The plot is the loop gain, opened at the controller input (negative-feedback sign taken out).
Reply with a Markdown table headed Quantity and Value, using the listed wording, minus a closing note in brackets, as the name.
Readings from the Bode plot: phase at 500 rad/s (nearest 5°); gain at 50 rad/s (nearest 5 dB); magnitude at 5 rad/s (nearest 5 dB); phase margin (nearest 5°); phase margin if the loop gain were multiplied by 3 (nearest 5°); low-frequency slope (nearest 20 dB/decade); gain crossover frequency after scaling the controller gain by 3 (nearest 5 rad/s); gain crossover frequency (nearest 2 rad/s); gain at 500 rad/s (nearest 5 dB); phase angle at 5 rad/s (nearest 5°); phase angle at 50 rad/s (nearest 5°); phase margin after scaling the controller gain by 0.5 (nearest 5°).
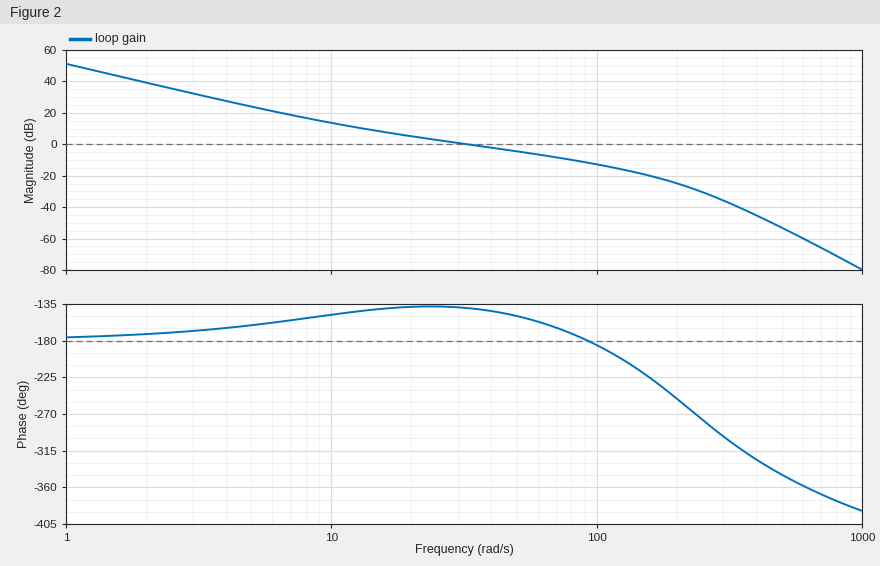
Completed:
| Quantity | Value |
|---|---|
| phase at 500 rad/s | -345° |
| gain at 50 rad/s | -5 dB |
| magnitude at 5 rad/s | 25 dB |
| phase margin | 40° |
| phase margin if the loop gain were multiplied by 3 | 10° |
| low-frequency slope | -40 dB/decade |
| gain crossover frequency after scaling the controller gain by 3 | 80 rad/s |
| gain crossover frequency | 32 rad/s |
| gain at 500 rad/s | -55 dB |
| phase angle at 5 rad/s | -160° |
| phase angle at 50 rad/s | -150° |
| phase margin after scaling the controller gain by 0.5 | 40° |
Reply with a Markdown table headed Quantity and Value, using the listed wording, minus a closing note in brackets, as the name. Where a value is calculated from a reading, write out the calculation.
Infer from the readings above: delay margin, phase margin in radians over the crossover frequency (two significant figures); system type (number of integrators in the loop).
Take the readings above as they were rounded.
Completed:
| Quantity | Value |
|---|---|
| delay margin, phase margin in radians over the crossover frequency | 40 × π / 180 / 32 = 0.022 s |
| system type | 2 |
